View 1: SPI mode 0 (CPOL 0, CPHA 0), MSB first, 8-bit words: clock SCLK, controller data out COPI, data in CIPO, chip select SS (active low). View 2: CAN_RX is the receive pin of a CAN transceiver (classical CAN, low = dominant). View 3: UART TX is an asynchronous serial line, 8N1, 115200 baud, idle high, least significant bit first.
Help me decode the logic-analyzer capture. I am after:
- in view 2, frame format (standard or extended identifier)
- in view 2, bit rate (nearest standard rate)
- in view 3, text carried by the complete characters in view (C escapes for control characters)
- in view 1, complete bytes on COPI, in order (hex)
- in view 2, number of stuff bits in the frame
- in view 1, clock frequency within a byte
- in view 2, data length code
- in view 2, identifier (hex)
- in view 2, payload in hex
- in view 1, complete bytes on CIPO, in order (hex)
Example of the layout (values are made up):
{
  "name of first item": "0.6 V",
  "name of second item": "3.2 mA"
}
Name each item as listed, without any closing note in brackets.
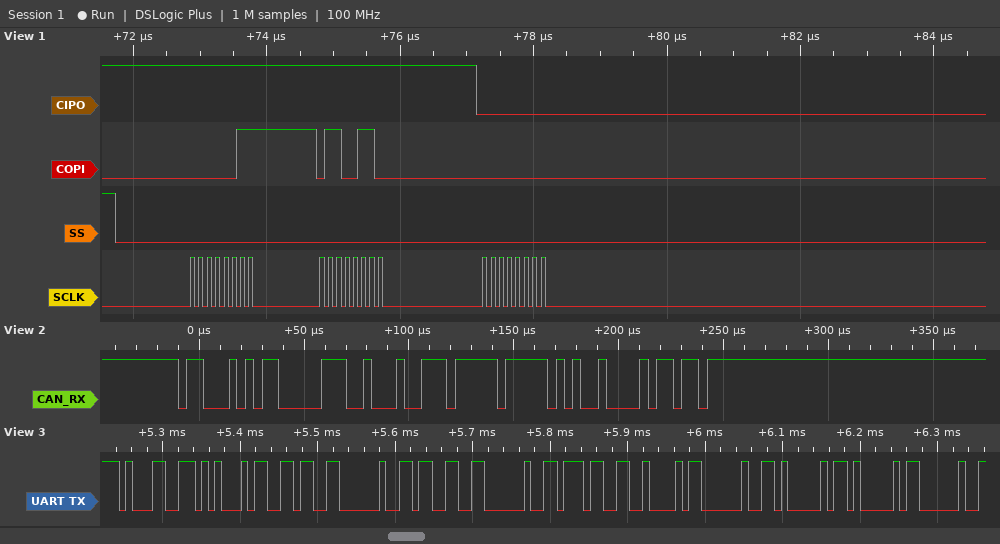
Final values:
{
  "in view 2, frame format": "standard",
  "in view 2, bit rate": "250 kbit/s",
  "in view 3, text carried by the complete characters in view": "\"1E6 3 7B AA \"",
  "in view 1, complete bytes on COPI, in order": "03 66 00",
  "in view 2, number of stuff bits in the frame": "3",
  "in view 1, clock frequency within a byte": "8 MHz",
  "in view 2, data length code": "3",
  "in view 2, identifier": "0x62B",
  "in view 2, payload in hex": "22 77 FF",
  "in view 1, complete bytes on CIPO, in order": "FF FF 00"
}
